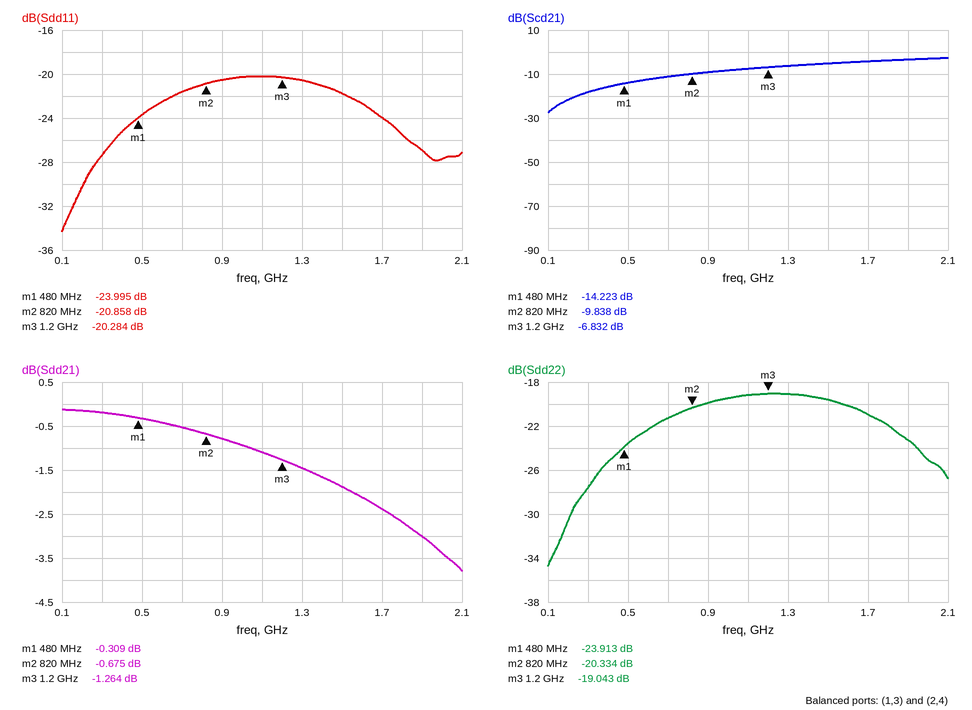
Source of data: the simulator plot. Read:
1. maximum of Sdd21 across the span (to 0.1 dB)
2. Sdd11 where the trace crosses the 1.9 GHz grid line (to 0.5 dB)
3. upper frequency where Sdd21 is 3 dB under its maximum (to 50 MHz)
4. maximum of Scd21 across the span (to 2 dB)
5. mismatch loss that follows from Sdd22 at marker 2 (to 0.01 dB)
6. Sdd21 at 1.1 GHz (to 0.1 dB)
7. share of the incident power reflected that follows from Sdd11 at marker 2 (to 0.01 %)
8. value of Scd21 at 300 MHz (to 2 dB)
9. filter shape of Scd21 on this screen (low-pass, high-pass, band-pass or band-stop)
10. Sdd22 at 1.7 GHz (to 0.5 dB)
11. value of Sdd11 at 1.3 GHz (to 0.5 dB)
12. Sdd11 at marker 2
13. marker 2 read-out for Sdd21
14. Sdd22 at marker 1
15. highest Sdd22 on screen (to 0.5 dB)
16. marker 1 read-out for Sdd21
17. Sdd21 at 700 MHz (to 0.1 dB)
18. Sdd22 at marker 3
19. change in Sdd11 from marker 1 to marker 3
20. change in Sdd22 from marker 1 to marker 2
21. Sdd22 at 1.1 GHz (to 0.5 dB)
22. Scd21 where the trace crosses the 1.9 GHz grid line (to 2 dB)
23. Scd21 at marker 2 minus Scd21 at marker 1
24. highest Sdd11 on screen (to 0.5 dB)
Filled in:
-0.1 dB
-27.0 dB
1.95 GHz
-2 dB
0.04 dB
-1.1 dB
0.82 %
-18 dB
high-pass
-21.0 dB
-20.5 dB
-20.858 dB
-0.675 dB
-23.913 dB
-19.0 dB
-0.309 dB
-0.5 dB
-19.043 dB
3.711 dB
3.579 dB
-19.0 dB
-4 dB
4.385 dB
-20.0 dB
